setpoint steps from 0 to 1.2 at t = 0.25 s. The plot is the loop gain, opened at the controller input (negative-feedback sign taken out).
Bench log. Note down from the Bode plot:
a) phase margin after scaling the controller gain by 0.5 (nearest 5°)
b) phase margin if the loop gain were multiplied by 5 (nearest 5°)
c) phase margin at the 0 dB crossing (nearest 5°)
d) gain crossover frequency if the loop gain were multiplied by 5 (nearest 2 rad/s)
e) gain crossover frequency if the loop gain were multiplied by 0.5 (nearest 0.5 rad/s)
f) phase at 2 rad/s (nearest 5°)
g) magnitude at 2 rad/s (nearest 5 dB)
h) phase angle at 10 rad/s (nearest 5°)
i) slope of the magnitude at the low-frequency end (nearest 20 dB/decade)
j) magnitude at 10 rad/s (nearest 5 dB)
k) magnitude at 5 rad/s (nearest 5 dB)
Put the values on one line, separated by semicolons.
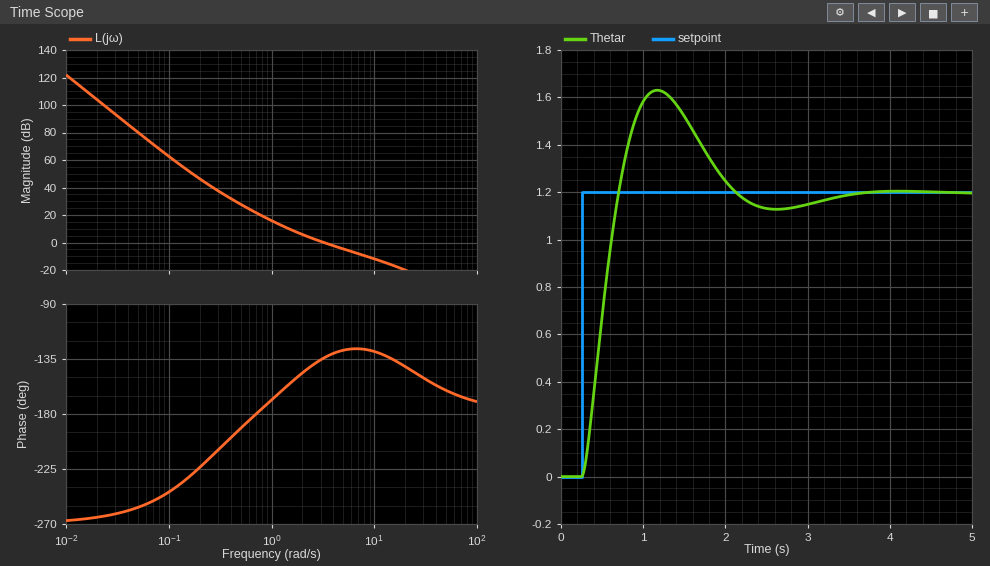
35°; 50°; 45°; 12 rad/s; 2.0 rad/s; -145°; 5 dB; -130°; -60 dB/decade; -10 dB; -5 dB
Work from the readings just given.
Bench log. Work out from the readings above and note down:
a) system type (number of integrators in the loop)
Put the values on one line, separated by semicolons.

3
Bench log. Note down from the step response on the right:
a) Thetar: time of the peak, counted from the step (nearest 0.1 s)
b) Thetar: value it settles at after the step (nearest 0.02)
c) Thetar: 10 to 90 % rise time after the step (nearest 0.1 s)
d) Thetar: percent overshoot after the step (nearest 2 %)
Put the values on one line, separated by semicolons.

0.9 s; 1.20; 0.3 s; 36 %
